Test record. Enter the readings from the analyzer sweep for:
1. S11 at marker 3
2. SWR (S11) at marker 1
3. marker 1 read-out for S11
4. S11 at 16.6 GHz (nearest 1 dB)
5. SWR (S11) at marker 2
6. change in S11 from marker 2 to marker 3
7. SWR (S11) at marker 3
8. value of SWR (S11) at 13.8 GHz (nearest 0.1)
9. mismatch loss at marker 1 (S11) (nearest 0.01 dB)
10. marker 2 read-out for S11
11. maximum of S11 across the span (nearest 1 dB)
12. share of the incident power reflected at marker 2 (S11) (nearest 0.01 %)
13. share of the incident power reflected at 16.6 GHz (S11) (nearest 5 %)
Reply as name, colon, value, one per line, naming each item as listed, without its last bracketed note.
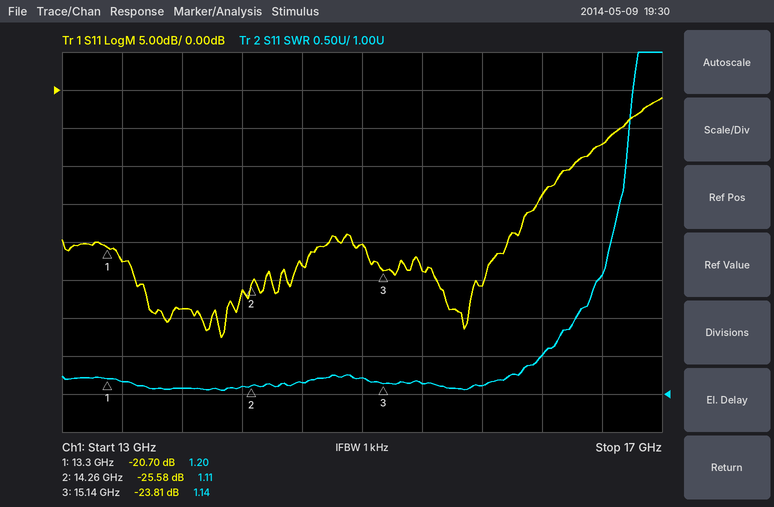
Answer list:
S11 at marker 3: -23.81 dB
SWR (S11) at marker 1: 1.20
marker 1 read-out for S11: -20.70 dB
S11 at 16.6 GHz: -7 dB
SWR (S11) at marker 2: 1.11
change in S11 from marker 2 to marker 3: 1.77 dB
SWR (S11) at marker 3: 1.14
value of SWR (S11) at 13.8 GHz: 1.1
mismatch loss at marker 1 (S11): 0.04 dB
marker 2 read-out for S11: -25.58 dB
maximum of S11 across the span: -1 dB
share of the incident power reflected at marker 2 (S11): 0.28 %
share of the incident power reflected at 16.6 GHz (S11): 20 %
